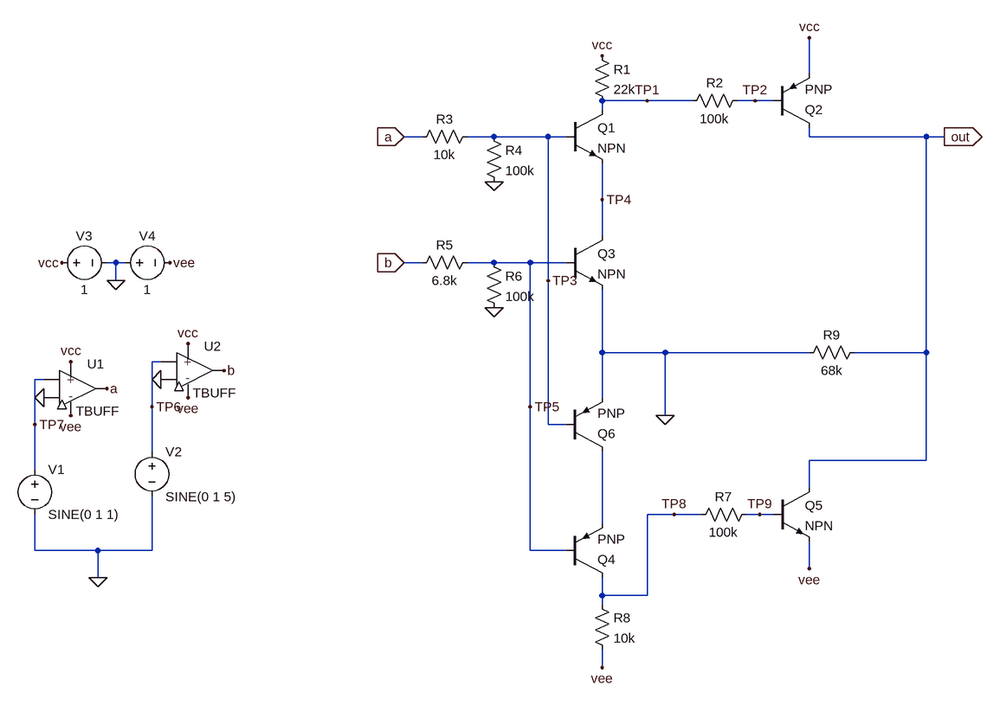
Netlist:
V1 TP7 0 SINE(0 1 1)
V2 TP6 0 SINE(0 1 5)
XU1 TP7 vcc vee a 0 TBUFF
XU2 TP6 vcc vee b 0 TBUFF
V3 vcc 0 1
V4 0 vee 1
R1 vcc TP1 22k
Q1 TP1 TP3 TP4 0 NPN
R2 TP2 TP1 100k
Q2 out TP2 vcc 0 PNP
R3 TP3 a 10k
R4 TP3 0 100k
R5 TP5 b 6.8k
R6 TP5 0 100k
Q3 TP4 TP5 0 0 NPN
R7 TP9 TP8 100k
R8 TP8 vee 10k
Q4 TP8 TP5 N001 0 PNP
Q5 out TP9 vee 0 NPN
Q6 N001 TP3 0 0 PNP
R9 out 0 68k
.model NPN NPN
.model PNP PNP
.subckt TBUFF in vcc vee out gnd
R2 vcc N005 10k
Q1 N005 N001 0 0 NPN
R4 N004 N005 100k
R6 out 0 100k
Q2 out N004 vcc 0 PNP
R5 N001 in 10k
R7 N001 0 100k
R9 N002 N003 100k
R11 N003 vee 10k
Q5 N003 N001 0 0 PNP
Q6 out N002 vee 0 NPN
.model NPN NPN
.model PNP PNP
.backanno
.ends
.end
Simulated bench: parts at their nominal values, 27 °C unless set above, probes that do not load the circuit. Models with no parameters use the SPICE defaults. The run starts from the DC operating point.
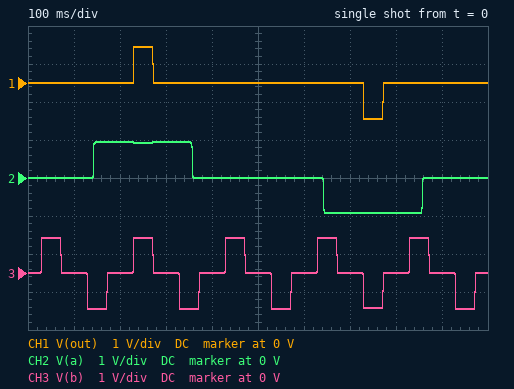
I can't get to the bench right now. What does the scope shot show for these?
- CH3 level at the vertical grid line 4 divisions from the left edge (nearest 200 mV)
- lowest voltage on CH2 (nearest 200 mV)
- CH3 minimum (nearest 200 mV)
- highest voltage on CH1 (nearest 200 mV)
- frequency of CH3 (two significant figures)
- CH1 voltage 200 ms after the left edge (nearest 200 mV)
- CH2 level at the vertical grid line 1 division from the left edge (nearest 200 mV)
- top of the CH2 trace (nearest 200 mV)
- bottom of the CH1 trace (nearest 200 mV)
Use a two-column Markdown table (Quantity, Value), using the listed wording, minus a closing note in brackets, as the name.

| Quantity | Value |
|---|---|
| CH3 level at the vertical grid line 4 divisions from the left edge | 0 V |
| lowest voltage on CH2 | -1.0 V |
| CH3 minimum | -1.0 V |
| highest voltage on CH1 | 1.0 V |
| frequency of CH3 | 5.0 Hz |
| CH1 voltage 200 ms after the left edge | 0 V |
| CH2 level at the vertical grid line 1 division from the left edge | 0 V |
| top of the CH2 trace | 1.0 V |
| bottom of the CH1 trace | -1.0 V |
